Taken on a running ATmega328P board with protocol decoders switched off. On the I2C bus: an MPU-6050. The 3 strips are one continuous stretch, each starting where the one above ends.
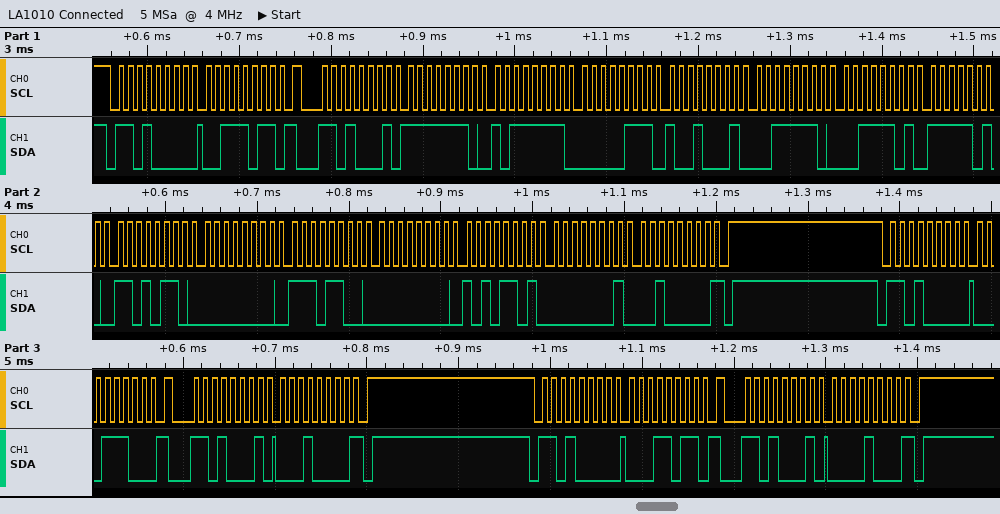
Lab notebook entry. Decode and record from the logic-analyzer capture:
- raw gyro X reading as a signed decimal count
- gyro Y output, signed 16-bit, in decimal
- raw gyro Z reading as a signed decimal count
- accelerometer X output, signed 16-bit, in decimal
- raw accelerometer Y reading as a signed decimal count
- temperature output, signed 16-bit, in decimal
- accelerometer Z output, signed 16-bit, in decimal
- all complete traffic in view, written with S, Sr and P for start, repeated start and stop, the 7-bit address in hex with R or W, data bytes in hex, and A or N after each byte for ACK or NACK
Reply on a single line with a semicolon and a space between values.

236; 173; 288; -321; 1937; -1322; 15933; S 68W A 3B A Sr 68R A FE A BF A 07 A 91 A 3E A 3D A FA A D6 A 00 A EC A 00 A AD A 01 A 20 N P S 68W A 1C A Sr 68R A 10 N P S 68W A 1B A Sr 68R A 08 N P
